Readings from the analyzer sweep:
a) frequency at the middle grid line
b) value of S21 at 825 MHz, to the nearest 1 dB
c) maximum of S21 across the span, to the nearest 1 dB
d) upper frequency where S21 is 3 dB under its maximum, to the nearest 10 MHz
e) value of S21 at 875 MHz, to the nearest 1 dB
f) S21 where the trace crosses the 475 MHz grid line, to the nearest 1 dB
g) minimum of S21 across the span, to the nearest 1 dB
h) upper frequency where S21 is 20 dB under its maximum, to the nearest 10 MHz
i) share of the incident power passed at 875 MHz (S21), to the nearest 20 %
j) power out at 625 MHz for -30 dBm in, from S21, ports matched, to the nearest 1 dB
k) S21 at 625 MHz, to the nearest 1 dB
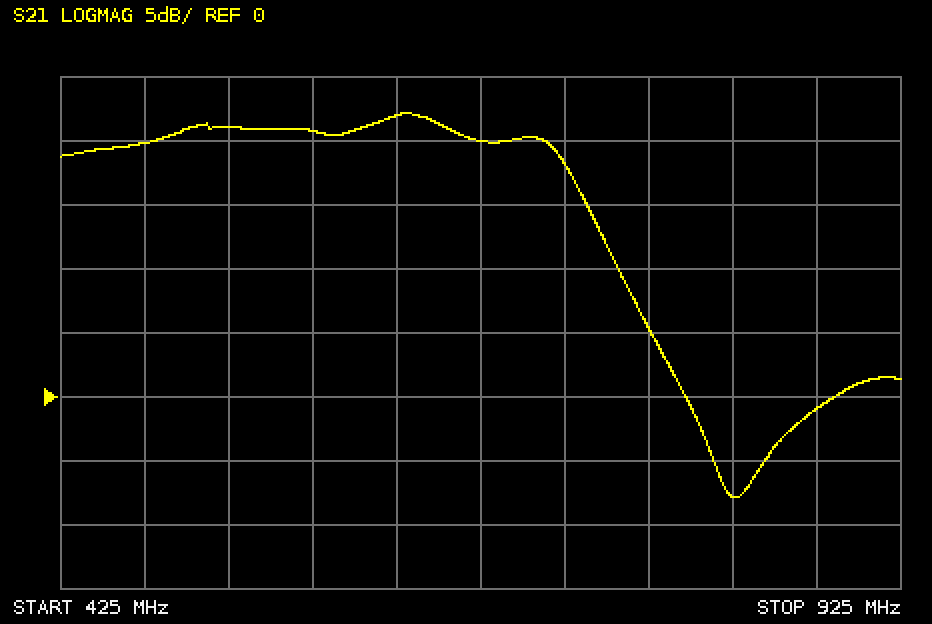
675 MHz
-8 dB
22 dB
720 MHz
-1 dB
20 dB
-8 dB
790 MHz
80 %
-8 dBm
22 dB
